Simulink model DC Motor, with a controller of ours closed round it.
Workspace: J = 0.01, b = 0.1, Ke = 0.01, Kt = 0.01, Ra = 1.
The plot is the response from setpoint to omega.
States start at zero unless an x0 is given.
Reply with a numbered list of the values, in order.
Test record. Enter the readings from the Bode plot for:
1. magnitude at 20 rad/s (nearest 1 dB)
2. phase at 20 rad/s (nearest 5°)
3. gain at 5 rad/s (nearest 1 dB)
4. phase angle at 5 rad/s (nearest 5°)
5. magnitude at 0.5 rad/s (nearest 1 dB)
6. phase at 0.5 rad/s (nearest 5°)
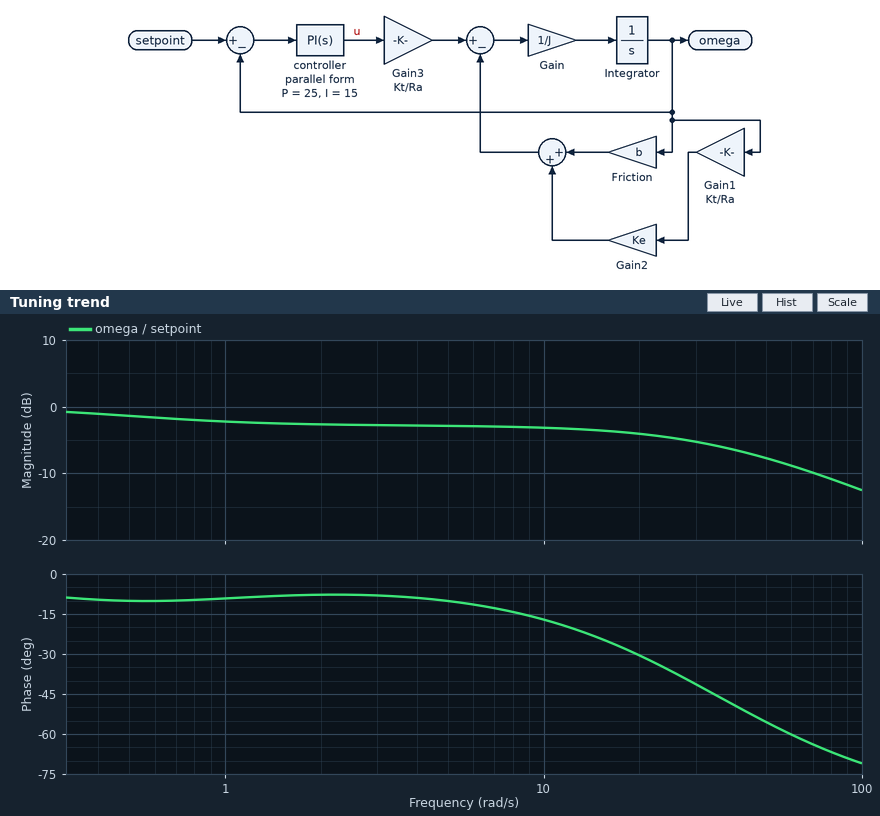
1. -4 dB
2. -30°
3. -3 dB
4. -10°
5. -1 dB
6. -10°
